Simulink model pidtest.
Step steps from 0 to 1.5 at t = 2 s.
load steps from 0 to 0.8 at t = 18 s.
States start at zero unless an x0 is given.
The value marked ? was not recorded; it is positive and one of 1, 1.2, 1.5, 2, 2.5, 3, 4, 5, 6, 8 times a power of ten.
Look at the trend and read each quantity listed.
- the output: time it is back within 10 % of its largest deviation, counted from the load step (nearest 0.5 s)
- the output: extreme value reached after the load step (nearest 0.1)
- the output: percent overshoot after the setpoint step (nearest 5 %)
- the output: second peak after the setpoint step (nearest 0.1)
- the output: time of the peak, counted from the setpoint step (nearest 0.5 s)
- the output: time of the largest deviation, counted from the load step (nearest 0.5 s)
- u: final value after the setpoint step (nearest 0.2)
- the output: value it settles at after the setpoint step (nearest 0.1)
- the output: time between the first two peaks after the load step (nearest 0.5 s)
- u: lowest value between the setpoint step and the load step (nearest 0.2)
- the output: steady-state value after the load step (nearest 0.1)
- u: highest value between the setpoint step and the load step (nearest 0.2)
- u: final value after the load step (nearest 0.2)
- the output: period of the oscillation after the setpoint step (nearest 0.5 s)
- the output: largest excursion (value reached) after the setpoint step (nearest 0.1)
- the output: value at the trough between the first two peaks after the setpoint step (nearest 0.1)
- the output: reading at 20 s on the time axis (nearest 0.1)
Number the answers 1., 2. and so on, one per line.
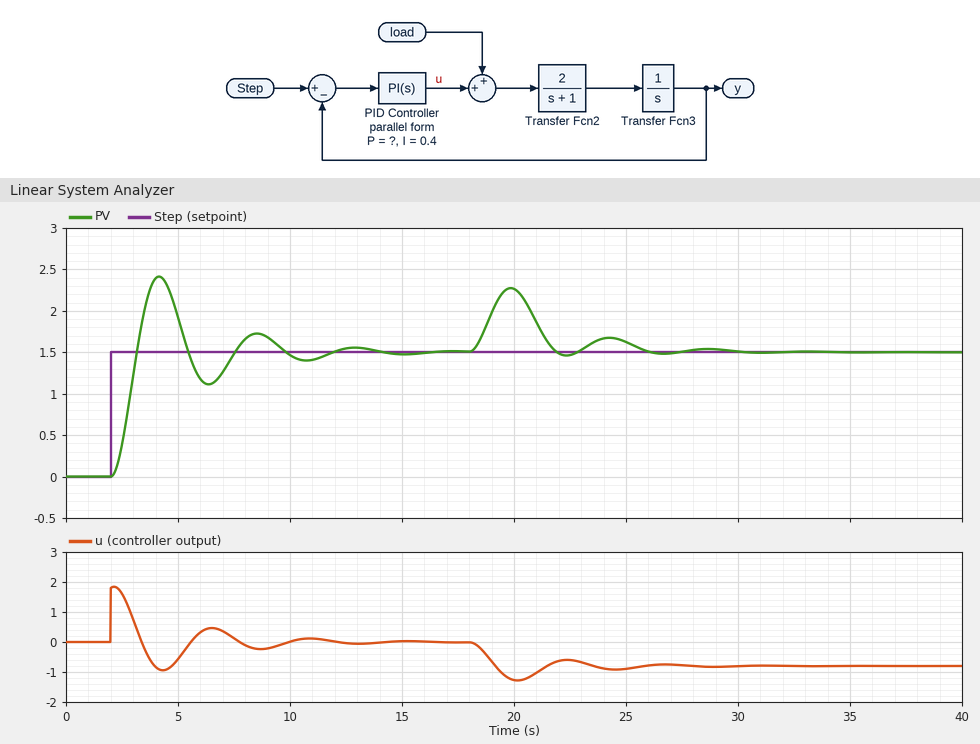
1. 7.5 s
2. 2.3
3. 60 %
4. 1.7
5. 2.0 s
6. 2.0 s
7. 0.0
8. 1.5
9. 4.5 s
10. -1.0
11. 1.5
12. 1.8
13. -0.8
14. 4.5 s
15. 2.4
16. 1.1
17. 2.3
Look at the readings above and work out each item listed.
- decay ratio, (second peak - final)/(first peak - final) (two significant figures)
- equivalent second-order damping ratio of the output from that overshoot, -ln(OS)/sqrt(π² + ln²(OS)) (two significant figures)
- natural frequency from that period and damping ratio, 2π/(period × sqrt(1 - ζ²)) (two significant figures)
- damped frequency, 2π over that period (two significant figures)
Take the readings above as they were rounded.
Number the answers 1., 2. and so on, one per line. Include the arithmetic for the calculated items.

1. (1.7 - 1.5) / (2.4 - 1.5) = 0.22
2. ln(0.6) = -0.511; 0.511 / sqrt(9.870 + 0.261) = 0.16
3. 2π / (4.5 × sqrt(1 - 0.16²)) = 1.4 rad/s
4. 2π / 4.5 = 1.4 rad/s
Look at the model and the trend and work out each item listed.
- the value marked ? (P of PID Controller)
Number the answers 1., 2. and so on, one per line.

1. 1.2
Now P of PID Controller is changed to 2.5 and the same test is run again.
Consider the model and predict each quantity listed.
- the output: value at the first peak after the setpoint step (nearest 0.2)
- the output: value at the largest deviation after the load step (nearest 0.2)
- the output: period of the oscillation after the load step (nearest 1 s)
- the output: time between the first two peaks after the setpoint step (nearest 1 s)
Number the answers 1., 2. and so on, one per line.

1. 2.4
2. 2.0
3. 3 s
4. 3 s
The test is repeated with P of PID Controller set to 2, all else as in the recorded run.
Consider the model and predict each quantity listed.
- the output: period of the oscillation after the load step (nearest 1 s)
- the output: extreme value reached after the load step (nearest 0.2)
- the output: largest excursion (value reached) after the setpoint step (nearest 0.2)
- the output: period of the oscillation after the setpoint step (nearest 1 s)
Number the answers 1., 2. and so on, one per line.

1. 3 s
2. 2.0
3. 2.4
4. 3 s
